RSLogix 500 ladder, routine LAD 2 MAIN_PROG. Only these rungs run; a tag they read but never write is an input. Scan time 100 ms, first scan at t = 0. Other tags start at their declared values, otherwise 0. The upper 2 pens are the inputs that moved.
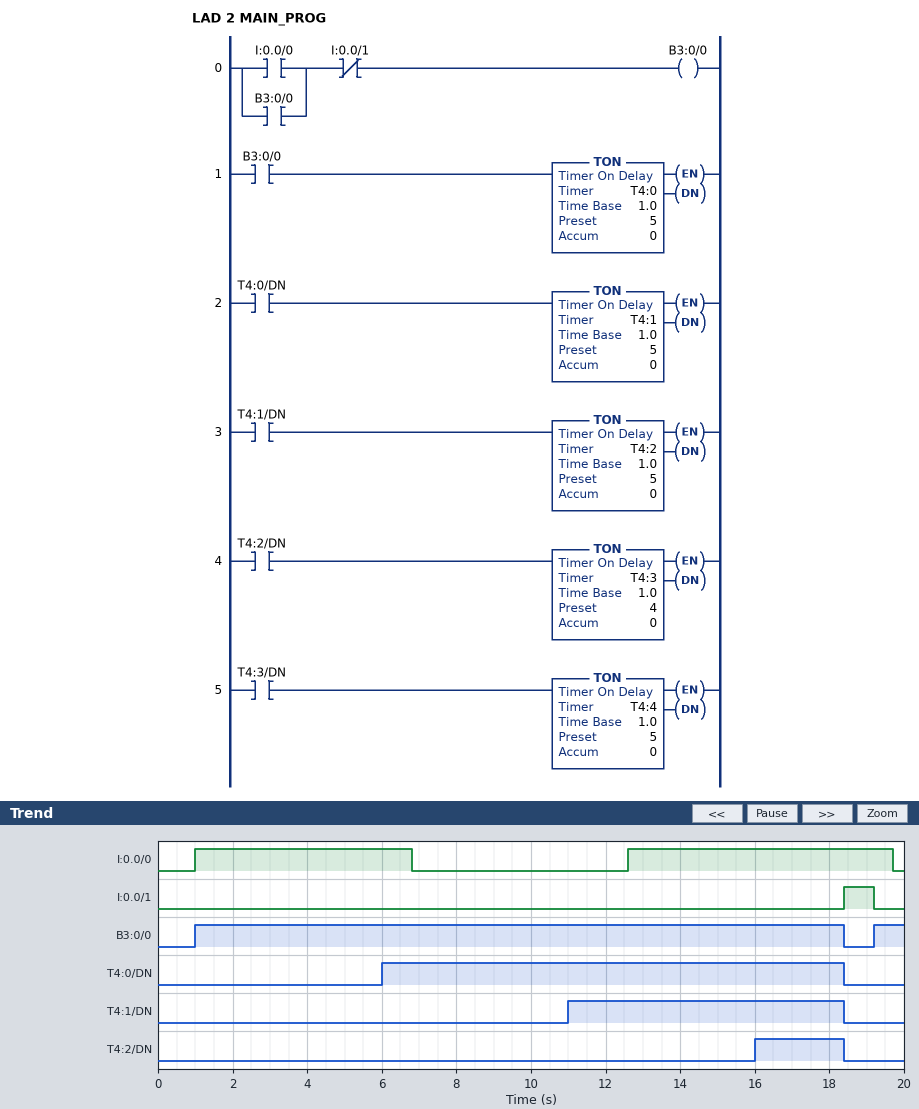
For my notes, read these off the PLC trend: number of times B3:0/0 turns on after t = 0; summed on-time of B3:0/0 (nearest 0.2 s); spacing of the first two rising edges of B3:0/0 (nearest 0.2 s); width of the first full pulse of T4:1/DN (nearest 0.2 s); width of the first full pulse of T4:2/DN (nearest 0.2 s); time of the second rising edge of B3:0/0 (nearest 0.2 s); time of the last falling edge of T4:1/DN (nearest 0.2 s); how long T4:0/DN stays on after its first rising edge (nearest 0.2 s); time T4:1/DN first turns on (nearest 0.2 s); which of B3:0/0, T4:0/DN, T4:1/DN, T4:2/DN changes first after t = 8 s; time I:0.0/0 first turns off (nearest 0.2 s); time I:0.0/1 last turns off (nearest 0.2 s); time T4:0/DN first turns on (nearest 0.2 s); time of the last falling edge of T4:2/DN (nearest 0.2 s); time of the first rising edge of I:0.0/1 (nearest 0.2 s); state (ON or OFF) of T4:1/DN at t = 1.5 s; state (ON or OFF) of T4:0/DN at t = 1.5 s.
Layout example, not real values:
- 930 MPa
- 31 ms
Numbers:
- 2
- 18.2 s
- 18.2 s
- 7.4 s
- 2.4 s
- 19.2 s
- 18.4 s
- 12.4 s
- 11.0 s
- T4:1/DN
- 6.8 s
- 19.2 s
- 6.0 s
- 18.4 s
- 18.4 s
- OFF
- OFF
